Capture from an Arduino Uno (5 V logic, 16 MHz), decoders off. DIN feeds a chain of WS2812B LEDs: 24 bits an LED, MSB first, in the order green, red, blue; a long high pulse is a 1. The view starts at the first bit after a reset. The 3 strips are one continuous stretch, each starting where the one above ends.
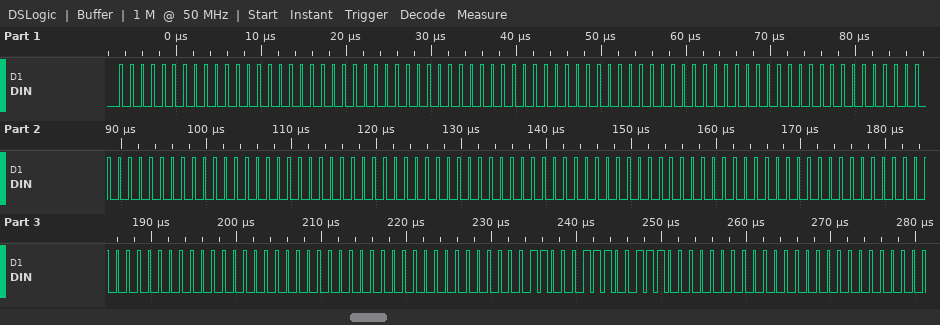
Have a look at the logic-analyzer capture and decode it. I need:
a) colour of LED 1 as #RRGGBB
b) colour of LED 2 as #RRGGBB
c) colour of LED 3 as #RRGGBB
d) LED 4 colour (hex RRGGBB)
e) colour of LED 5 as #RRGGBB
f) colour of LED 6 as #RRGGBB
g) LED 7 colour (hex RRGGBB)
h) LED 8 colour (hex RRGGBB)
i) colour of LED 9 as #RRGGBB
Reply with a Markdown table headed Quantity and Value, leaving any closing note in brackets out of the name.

| Quantity | Value |
|---|---|
| colour of LED 1 as #RRGGBB | #000000 |
| colour of LED 2 as #RRGGBB | #000000 |
| colour of LED 3 as #RRGGBB | #000000 |
| LED 4 colour | #000000 |
| colour of LED 5 as #RRGGBB | #000000 |
| colour of LED 6 as #RRGGBB | #000000 |
| LED 7 colour | #000000 |
| LED 8 colour | #000000 |
| colour of LED 9 as #RRGGBB | #9C6300 |
